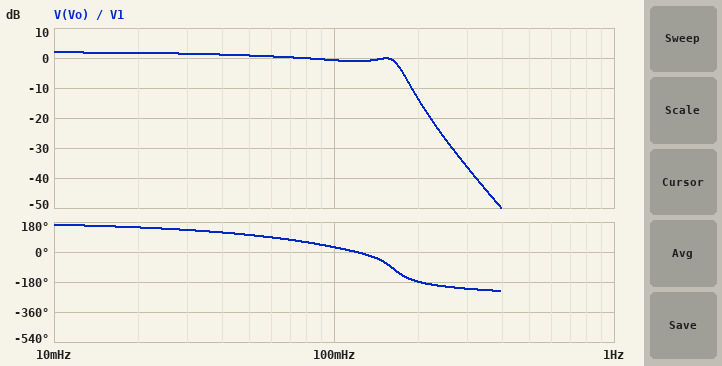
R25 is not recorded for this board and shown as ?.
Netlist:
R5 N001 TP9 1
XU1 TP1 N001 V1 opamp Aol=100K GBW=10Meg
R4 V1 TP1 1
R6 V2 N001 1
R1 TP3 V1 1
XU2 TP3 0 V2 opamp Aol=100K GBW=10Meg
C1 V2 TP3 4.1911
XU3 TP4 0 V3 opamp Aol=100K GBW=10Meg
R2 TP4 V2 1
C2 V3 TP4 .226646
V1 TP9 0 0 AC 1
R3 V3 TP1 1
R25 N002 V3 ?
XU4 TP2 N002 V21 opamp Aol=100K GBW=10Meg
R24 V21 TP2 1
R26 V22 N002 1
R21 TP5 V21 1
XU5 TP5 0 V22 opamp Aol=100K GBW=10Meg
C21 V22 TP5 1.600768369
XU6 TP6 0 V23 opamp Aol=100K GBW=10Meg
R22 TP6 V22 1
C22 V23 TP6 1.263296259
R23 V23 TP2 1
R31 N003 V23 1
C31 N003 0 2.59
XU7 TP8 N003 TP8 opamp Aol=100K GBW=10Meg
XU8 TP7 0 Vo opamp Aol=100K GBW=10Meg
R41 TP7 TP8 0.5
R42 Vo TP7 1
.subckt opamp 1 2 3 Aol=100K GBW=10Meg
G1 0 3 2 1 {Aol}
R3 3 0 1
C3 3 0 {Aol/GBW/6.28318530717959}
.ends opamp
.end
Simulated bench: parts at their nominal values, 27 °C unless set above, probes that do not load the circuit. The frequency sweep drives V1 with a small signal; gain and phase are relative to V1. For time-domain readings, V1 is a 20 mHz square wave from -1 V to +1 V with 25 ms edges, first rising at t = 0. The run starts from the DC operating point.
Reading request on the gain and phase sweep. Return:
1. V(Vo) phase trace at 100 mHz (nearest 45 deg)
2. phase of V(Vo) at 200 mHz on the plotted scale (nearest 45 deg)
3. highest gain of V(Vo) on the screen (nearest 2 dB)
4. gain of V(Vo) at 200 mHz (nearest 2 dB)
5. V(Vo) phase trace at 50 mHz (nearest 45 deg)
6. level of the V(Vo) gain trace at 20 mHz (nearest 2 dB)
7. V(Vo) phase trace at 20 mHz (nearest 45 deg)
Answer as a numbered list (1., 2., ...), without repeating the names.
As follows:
1. 45 deg
2. -180 deg
3. 2 dB
4. -14 dB
5. 90 deg
6. 2 dB
7. 135 deg
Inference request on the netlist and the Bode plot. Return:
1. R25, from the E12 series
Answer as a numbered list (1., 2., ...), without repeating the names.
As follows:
1. 2.2 Ω
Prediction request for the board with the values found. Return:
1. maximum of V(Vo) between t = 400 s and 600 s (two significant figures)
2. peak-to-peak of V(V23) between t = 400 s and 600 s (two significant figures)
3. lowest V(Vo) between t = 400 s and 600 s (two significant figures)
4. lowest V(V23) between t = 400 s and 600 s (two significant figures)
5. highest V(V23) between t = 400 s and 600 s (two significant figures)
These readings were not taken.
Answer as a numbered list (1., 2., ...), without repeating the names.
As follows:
1. 1.3 V
2. 2.3 V
3. -1.3 V
4. -1.1 V
5. 1.1 V
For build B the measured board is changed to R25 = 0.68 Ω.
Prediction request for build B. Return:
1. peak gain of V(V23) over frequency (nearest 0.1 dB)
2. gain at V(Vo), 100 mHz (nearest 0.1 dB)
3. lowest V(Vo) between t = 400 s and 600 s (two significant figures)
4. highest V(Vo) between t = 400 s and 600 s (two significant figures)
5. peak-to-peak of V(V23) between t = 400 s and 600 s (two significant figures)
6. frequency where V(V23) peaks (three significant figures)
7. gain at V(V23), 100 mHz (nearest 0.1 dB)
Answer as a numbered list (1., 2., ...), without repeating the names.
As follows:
1. 11.2 dB
2. 9.2 dB
3. -3.4 V
4. 3.4 V
5. 6.0 V
6. 154 mHz
7. 8.8 dB
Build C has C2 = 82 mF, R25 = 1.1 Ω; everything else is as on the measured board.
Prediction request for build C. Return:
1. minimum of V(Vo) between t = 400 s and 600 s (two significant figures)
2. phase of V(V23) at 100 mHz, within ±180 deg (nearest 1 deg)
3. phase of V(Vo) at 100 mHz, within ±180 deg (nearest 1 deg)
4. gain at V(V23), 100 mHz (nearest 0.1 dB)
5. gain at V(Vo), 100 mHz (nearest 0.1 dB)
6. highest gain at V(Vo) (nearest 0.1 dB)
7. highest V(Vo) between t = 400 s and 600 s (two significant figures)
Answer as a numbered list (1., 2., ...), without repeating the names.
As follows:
1. -2.0 V
2. -80 deg
3. 42 deg
4. 2.2 dB
5. 2.6 dB
6. 5.6 dB
7. 2.0 V
